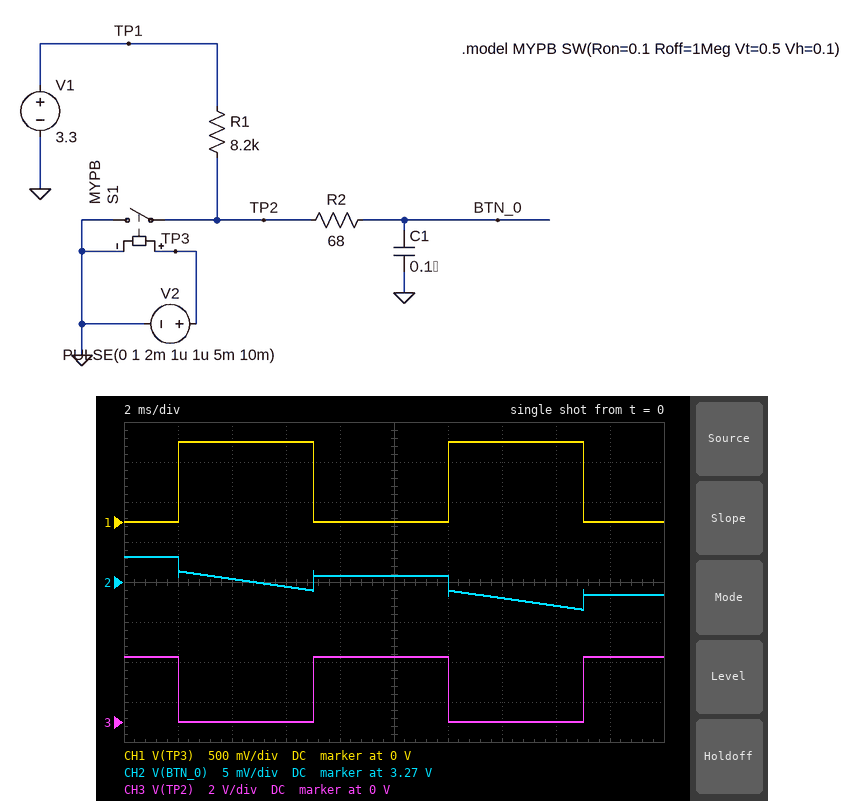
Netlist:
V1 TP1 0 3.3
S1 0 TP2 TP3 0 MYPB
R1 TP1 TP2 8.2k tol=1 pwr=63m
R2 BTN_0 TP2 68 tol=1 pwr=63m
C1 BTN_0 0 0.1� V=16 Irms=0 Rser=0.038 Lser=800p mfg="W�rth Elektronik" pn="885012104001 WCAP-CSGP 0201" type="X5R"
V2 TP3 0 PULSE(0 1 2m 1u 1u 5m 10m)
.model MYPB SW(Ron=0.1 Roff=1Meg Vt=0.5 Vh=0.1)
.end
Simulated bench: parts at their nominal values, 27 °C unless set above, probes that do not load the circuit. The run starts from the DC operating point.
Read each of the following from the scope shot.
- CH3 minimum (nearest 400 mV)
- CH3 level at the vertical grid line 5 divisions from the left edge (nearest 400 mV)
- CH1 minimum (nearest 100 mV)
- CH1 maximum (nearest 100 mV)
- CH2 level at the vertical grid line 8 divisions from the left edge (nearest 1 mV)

0 V
3.2 V
0 V
1.0 V
3.267 V
